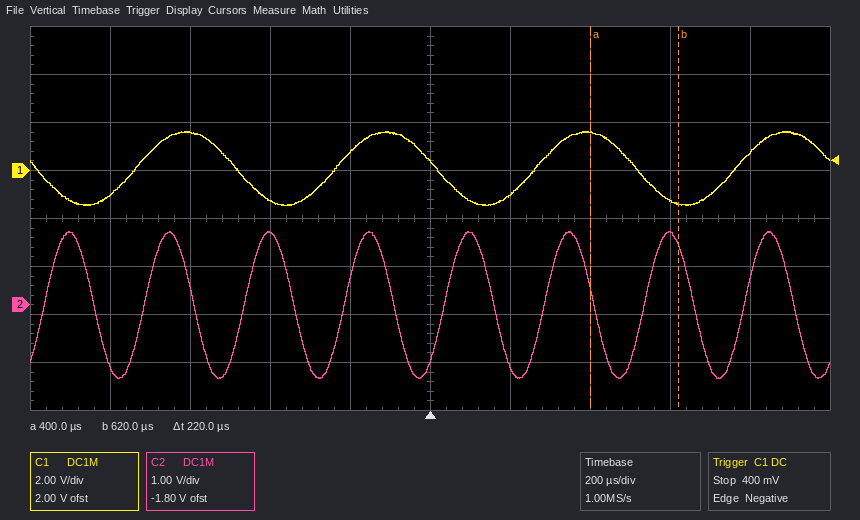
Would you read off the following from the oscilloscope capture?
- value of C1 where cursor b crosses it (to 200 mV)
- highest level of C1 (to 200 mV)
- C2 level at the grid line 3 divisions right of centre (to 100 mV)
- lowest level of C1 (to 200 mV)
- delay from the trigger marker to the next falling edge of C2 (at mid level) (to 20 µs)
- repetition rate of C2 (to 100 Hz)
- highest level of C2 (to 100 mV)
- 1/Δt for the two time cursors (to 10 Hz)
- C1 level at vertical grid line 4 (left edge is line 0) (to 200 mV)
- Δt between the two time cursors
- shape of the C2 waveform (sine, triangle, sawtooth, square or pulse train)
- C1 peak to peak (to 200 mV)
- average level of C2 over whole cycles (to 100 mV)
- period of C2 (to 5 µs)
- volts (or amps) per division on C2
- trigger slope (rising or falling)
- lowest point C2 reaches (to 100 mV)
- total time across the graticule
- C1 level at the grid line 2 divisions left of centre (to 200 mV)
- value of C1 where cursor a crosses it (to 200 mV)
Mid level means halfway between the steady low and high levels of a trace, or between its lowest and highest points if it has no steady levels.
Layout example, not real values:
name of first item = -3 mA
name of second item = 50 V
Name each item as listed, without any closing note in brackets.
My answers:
value of C1 where cursor b crosses it = -1.4 V
highest level of C1 = 1.6 V
C2 level at the grid line 3 divisions right of centre = 1.5 V
lowest level of C1 = -1.4 V
delay from the trigger marker to the next falling edge of C2 (at mid level) = 160 µs
repetition rate of C2 = 4.0 kHz
highest level of C2 = 1.5 V
1/Δt for the two time cursors = 4.55 kHz
C1 level at vertical grid line 4 (left edge is line 0) = 800 mV
Δt between the two time cursors = 220 µs
shape of the C2 waveform = sine
C1 peak to peak = 3.0 V
average level of C2 over whole cycles = 0.0 V
period of C2 = 250 µs
volts (or amps) per division on C2 = 1 V
trigger slope = falling
lowest point C2 reaches = -1.5 V
total time across the graticule = 2 ms
C1 level at the grid line 2 divisions left of centre = -1.2 V
value of C1 where cursor a crosses it = 1.6 V
